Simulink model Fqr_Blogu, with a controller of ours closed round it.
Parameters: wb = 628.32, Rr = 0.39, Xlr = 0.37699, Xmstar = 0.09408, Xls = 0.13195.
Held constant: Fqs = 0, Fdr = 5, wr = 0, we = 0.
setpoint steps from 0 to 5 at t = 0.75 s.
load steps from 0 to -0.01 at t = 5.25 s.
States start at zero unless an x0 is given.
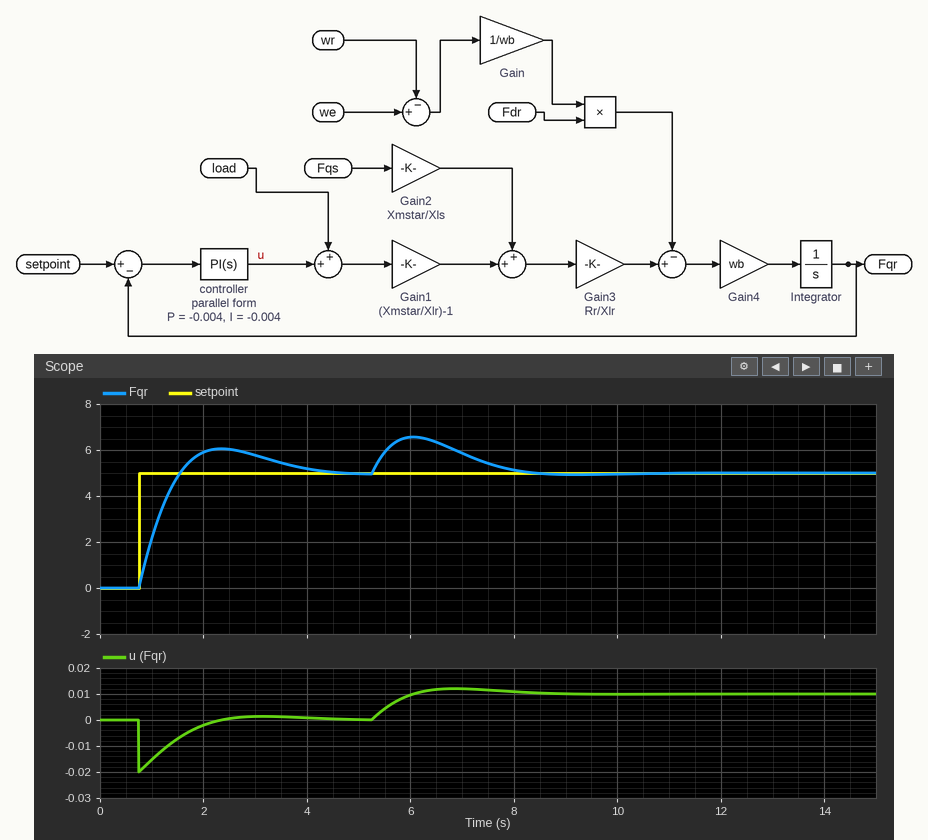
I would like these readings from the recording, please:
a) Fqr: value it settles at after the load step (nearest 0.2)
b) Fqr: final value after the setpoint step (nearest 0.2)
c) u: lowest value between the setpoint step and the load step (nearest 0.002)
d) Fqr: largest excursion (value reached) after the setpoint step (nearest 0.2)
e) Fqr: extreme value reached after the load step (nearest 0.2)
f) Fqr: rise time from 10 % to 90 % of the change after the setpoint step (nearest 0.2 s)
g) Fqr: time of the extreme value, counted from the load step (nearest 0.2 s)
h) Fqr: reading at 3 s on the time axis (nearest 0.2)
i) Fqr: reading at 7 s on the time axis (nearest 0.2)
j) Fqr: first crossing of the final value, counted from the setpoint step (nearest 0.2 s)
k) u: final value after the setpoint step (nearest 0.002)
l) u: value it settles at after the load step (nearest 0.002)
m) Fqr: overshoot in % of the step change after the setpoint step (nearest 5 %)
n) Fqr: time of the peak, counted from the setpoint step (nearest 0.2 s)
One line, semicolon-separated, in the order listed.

5.0; 5.0; -0.020; 6.0; 6.6; 0.6 s; 0.8 s; 5.8; 5.8; 0.8 s; 0.000; 0.010; 20 %; 1.6 s
